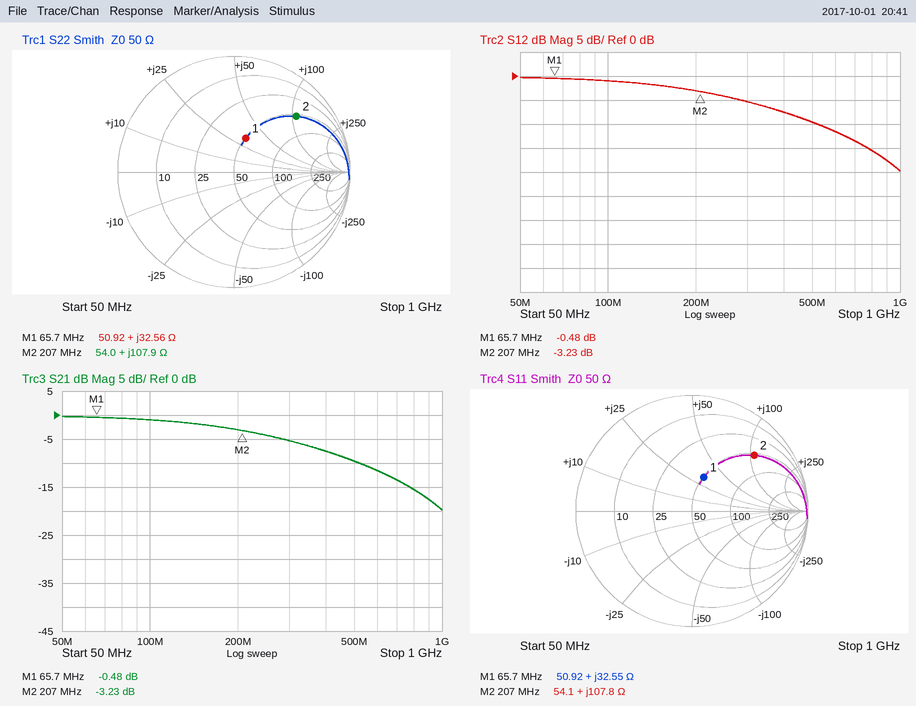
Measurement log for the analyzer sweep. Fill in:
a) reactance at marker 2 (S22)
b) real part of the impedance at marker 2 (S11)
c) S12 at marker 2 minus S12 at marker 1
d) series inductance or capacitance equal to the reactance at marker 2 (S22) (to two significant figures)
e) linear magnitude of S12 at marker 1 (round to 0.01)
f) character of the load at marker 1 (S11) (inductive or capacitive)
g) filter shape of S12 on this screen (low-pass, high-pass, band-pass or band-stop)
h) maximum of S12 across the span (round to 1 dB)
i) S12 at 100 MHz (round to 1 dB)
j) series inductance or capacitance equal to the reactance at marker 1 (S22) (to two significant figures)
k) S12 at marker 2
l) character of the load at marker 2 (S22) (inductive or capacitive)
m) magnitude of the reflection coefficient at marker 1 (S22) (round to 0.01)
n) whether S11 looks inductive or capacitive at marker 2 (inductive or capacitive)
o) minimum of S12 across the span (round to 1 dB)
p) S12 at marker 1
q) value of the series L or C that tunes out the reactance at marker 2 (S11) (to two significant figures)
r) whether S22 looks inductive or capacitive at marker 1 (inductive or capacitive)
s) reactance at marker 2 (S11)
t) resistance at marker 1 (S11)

+107.9 Ω
54.1 Ω
-2.75 dB
83 nH
0.95
inductive
low-pass
0 dB
-1 dB
79 nH
-3.23 dB
inductive
0.31
inductive
-20 dB
-0.48 dB
7.1 pF
inductive
+107.8 Ω
50.92 Ω
